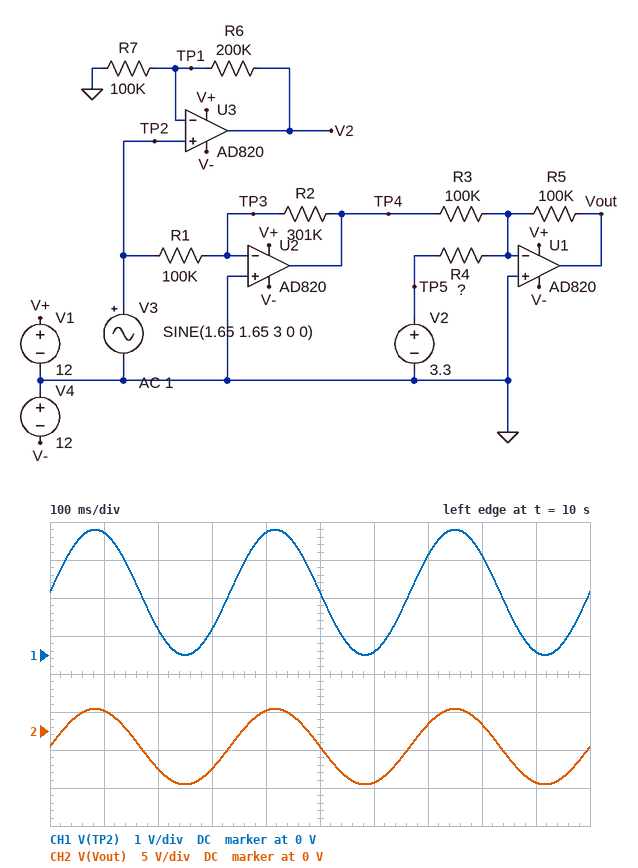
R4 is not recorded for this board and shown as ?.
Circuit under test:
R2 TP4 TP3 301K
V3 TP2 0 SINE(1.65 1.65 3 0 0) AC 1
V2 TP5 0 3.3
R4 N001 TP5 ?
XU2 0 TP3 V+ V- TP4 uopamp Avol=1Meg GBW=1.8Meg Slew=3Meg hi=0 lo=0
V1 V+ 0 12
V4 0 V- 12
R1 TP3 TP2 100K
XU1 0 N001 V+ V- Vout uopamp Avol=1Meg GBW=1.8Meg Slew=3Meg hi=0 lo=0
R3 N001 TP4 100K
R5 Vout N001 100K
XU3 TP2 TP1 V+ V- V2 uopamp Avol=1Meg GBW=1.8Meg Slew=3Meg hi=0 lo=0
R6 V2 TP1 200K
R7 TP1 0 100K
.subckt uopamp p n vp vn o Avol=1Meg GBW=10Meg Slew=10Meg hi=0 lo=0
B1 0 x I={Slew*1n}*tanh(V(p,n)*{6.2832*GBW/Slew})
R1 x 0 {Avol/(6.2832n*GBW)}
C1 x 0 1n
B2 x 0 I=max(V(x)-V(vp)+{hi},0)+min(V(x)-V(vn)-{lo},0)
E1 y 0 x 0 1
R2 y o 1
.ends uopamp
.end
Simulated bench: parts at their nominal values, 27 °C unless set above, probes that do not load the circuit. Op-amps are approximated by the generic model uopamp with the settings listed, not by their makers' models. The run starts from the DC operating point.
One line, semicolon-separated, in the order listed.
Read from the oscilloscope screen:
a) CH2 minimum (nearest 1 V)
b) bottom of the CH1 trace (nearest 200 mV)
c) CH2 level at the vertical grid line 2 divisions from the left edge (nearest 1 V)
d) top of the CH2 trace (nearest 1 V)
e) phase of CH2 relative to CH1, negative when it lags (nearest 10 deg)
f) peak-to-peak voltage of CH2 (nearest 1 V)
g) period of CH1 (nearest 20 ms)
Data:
-7 V; 0 V; -5 V; 3 V; 0 deg; 10 V; 340 ms
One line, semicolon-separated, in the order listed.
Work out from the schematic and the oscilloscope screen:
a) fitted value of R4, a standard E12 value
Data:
47 kΩ
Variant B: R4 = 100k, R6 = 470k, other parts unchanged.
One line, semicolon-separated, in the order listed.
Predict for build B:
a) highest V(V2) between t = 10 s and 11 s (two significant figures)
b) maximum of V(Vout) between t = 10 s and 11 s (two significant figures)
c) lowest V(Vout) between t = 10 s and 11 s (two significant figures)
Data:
12 V; 6.6 V; -3.3 V
